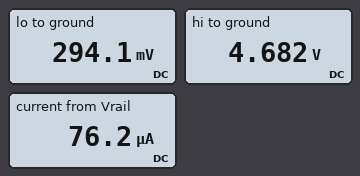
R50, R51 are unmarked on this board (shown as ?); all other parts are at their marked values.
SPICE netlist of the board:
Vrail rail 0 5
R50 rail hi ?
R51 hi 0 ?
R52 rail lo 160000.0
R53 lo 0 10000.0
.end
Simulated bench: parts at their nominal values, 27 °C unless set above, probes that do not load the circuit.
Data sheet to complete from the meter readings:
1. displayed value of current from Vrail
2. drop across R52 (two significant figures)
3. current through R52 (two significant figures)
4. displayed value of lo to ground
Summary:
76.2 µA
4.7 V
29 µA
294.1 mV
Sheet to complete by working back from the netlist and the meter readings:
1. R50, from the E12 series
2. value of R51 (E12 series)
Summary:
6.8 kΩ
100 kΩ
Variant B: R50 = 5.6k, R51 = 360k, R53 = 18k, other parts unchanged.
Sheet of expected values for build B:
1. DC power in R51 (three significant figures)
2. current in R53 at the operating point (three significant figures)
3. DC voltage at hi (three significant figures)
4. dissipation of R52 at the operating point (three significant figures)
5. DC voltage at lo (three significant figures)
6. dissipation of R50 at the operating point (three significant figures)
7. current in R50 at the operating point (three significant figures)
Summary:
67.3 µW
28.1 µA
4.92 V
126 µW
506 mV
1.05 µW
13.7 µA
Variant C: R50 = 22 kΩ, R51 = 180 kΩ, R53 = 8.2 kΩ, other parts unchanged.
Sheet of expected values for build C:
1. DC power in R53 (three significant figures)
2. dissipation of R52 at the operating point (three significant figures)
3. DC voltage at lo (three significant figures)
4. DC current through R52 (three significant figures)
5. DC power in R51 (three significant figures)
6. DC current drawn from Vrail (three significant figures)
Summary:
7.25 µW
141 µW
244 mV
29.7 µA
110 µW
54.5 µA
